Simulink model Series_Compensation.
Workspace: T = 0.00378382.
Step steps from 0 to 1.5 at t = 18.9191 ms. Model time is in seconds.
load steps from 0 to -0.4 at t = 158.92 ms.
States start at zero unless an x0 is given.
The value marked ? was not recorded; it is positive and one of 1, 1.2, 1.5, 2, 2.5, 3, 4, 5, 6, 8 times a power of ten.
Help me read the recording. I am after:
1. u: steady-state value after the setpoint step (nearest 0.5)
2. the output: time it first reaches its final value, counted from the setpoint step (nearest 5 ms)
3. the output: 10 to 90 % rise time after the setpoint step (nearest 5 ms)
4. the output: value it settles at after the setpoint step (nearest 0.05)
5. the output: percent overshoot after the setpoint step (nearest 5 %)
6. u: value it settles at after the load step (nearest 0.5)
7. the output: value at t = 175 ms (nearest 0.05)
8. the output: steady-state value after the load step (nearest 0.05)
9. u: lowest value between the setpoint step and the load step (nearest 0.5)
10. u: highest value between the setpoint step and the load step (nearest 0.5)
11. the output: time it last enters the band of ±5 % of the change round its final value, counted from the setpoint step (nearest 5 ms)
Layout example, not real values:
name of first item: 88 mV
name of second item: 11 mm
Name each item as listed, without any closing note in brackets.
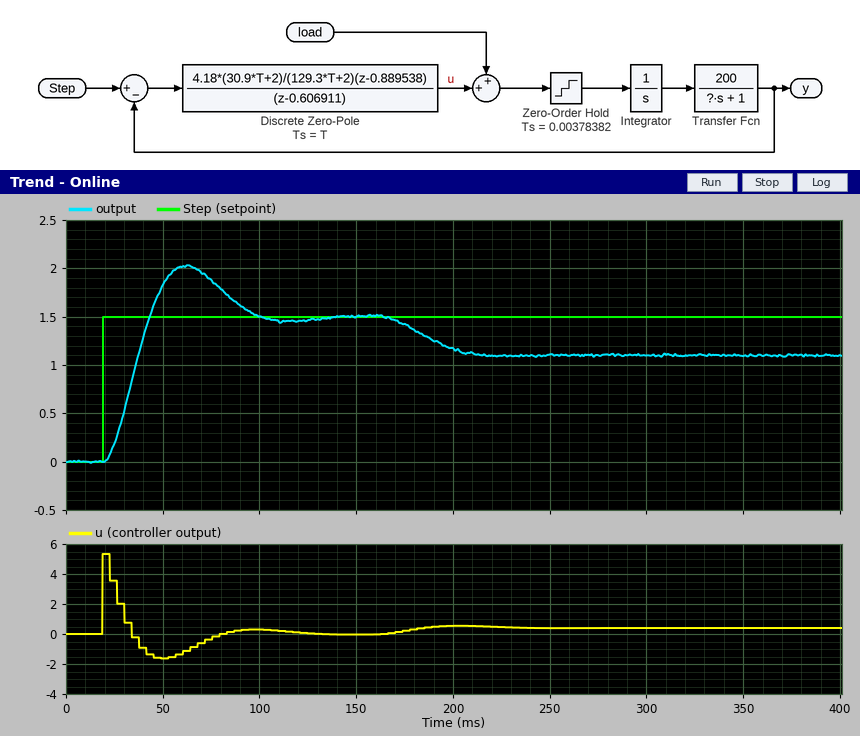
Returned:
u: steady-state value after the setpoint step: 0.0
the output: time it first reaches its final value, counted from the setpoint step: 25 ms
the output: 10 to 90 % rise time after the setpoint step: 15 ms
the output: value it settles at after the setpoint step: 1.50
the output: percent overshoot after the setpoint step: 35 %
u: value it settles at after the load step: 0.5
the output: value at t = 175 ms: 1.40
the output: steady-state value after the load step: 1.10
u: lowest value between the setpoint step and the load step: -1.5
u: highest value between the setpoint step and the load step: 5.5
the output: time it last enters the band of ±5 % of the change round its final value, counted from the setpoint step: 75 ms
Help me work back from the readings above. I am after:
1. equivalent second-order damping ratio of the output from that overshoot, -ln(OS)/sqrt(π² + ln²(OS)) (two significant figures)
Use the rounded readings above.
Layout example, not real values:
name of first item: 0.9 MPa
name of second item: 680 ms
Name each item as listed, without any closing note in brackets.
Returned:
equivalent second-order damping ratio of the output from that overshoot, -ln(OS)/sqrt(π² + ln²(OS)): 0.32
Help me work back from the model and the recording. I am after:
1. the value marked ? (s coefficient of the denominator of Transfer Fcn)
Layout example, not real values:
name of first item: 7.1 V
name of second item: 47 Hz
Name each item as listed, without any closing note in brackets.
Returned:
the value marked ?: 0.1
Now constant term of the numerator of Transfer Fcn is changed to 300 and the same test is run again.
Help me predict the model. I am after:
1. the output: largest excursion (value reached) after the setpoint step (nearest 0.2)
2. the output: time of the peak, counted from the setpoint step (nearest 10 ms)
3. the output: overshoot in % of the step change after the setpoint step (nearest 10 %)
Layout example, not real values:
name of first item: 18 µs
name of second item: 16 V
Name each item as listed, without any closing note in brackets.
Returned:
the output: largest excursion (value reached) after the setpoint step: 2.2
the output: time of the peak, counted from the setpoint step: 30 ms
the output: overshoot in % of the step change after the setpoint step: 40 %
